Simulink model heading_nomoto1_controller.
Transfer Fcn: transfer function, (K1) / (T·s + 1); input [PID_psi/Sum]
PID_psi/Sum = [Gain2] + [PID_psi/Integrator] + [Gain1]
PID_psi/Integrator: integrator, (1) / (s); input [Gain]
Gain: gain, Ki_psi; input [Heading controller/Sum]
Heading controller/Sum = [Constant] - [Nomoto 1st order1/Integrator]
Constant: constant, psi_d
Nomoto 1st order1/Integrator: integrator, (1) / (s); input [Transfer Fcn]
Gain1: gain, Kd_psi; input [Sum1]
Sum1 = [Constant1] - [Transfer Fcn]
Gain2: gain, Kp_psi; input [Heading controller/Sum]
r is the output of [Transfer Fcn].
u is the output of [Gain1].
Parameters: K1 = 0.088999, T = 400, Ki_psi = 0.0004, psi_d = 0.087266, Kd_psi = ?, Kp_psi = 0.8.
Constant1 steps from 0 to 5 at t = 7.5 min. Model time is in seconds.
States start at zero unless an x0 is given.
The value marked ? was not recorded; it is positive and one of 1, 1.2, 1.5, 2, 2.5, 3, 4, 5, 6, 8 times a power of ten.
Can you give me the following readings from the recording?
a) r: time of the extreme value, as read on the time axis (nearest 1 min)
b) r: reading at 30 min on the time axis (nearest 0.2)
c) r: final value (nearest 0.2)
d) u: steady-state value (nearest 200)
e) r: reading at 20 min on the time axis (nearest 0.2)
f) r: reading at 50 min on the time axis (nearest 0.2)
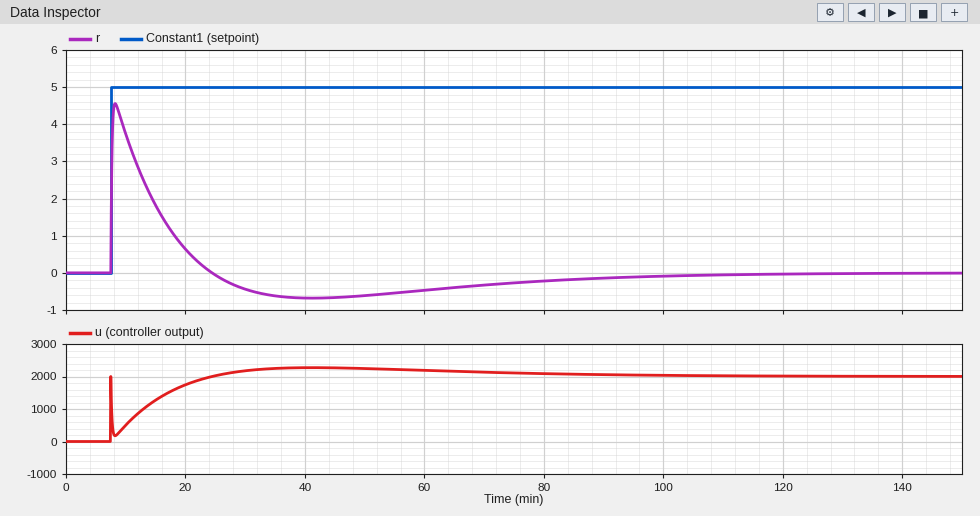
8 min
-0.4
0.0
2000
0.6
-0.6
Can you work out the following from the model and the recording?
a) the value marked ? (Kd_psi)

400
